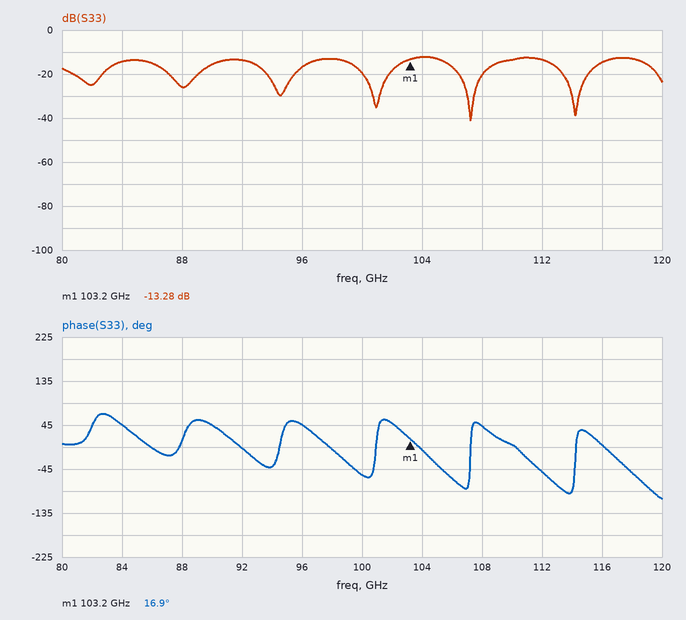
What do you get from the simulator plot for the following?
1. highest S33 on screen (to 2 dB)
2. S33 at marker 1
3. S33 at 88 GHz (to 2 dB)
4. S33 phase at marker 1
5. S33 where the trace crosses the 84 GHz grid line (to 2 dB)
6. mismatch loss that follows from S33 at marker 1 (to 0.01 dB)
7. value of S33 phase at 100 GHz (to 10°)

-12 dB
-13.28 dB
-26 dB
16.9°
-14 dB
0.21 dB
-60°
